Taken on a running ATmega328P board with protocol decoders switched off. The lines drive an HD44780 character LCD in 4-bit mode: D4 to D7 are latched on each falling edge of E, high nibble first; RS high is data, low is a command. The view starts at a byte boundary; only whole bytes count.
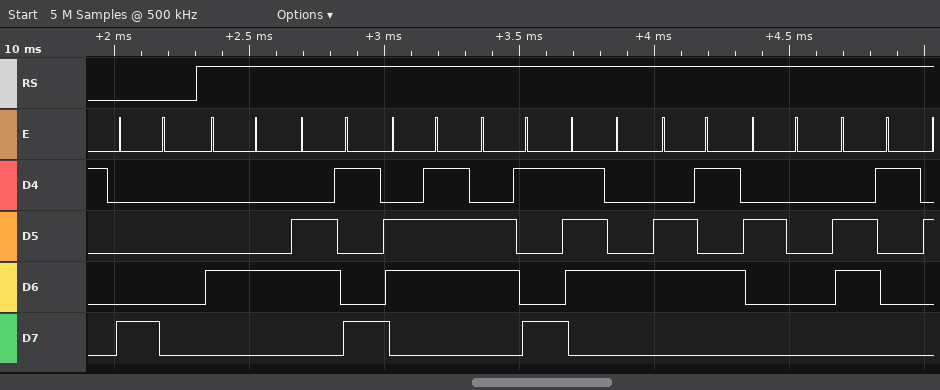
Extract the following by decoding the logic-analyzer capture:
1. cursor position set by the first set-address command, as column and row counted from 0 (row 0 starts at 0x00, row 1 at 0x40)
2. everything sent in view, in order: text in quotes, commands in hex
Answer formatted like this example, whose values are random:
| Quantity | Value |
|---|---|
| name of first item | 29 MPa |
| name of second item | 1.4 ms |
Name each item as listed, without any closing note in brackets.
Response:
| Quantity | Value |
|---|---|
| cursor position set by the first set-address command, as column and row counted from 0 | column 0, row 0 |
| everything sent in view, in order: text in quotes, commands in hex | 0x80 "Digite a" |
